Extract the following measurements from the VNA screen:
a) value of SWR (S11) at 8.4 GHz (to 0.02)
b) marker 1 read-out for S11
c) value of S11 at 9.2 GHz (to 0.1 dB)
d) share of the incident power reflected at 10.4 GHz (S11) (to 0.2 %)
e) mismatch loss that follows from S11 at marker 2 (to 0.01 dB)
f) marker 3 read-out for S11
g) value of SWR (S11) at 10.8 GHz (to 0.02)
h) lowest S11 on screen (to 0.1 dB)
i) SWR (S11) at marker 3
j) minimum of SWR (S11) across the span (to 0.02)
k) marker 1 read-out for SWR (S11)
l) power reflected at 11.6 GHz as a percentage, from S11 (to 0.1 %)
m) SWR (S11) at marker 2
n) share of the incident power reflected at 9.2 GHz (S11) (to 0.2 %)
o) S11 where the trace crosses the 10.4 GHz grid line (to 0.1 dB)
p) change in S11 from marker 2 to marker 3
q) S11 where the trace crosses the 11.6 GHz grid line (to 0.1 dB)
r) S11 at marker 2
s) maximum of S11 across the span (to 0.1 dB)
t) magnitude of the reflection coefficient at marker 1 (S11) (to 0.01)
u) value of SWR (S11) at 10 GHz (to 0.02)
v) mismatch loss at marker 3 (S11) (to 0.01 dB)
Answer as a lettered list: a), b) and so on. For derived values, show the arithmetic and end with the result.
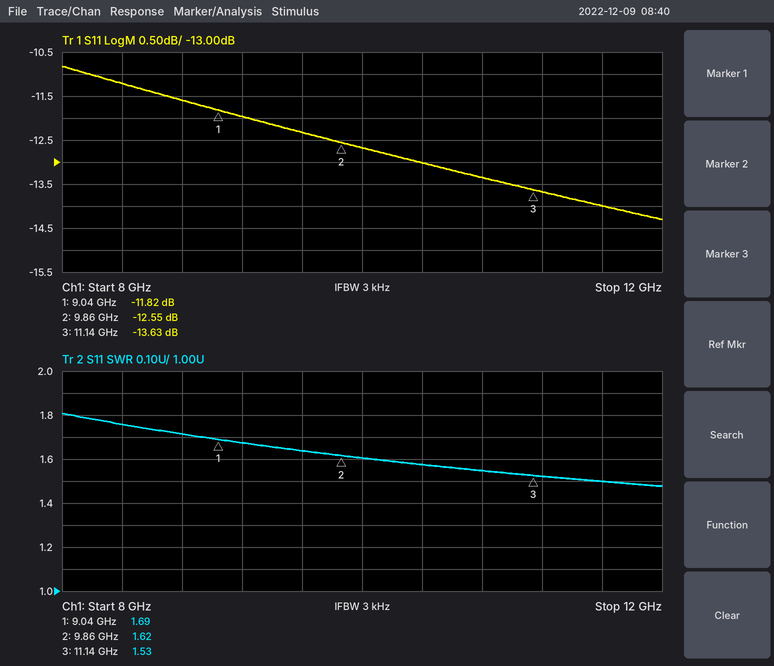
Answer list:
a) 1.76
b) -11.82 dB
c) -12.0 dB
d) 10^(-13/10) ≈ 5.0 %
e) −10 log10(1 − 10^(-12.55/10)) ≈ 0.25 dB
f) -13.63 dB
g) 1.54
h) -14.3 dB
i) 1.53
j) 1.48
k) 1.69
l) 10^(-14/10) ≈ 4.0 %
m) 1.62
n) 10^(-12/10) ≈ 6.31 %, so 6.4 % to the nearest 0.2 %
o) -13.0 dB
p) -13.63 − (-12.55) = -1.08 dB
q) -14.0 dB
r) -12.55 dB
s) -10.8 dB
t) 10^(-11.82/20) ≈ 0.26
u) 1.60
v) −10 log10(1 − 10^(-13.63/10)) ≈ 0.19 dB
